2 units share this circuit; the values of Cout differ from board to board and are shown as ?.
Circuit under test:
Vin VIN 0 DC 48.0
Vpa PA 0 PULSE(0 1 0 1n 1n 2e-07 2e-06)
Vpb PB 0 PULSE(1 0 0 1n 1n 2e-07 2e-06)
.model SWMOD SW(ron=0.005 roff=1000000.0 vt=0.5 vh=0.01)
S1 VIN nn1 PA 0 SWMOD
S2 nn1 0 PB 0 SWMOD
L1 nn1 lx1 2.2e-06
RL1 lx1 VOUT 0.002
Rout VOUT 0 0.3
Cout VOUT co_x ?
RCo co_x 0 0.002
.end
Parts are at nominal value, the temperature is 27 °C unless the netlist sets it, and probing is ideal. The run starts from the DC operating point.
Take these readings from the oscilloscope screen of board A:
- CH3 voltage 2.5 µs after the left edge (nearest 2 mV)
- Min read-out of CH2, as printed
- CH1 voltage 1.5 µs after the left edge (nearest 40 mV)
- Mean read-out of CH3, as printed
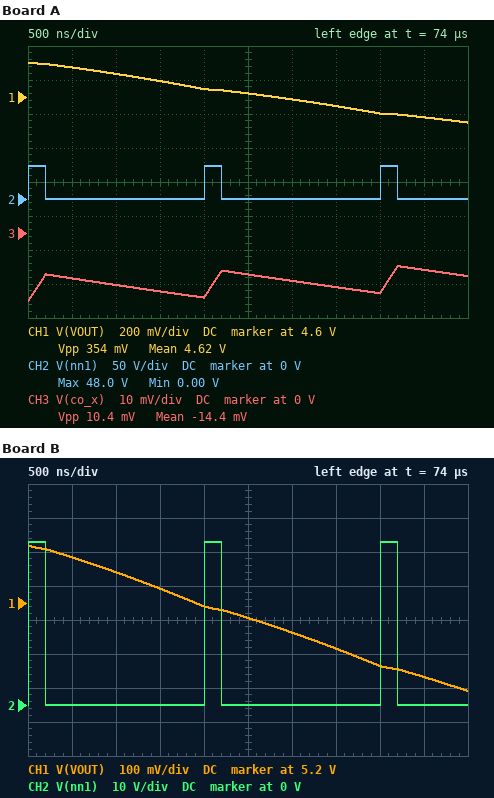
-12 mV
0.00 V
4.68 V
-14.4 mV
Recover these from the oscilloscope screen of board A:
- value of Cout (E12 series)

100 µF
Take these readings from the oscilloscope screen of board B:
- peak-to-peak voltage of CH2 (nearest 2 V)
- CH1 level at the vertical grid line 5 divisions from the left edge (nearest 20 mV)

48 V
5.16 V
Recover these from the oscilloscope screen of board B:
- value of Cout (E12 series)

120 µF
